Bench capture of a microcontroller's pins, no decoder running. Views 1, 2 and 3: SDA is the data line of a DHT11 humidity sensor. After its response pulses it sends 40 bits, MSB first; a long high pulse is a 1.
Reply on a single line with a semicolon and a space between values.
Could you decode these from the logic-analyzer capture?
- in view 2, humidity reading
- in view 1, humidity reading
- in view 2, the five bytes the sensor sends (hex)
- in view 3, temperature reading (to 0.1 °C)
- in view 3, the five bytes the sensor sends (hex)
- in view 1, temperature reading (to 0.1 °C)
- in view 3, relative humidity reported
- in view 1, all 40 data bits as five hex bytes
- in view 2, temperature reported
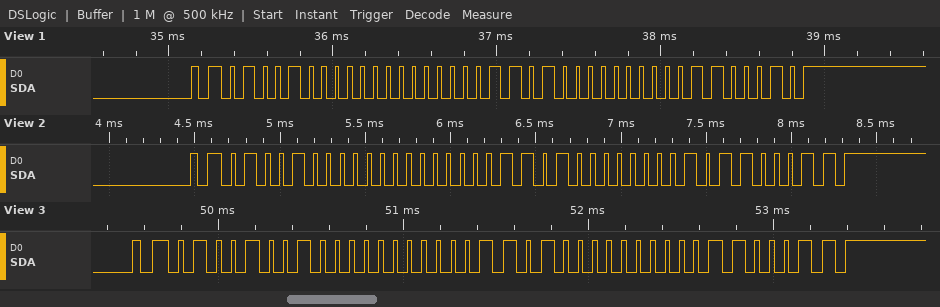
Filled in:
72 %; 72 %; 48 00 1A 01 63; 26.0 °C; 49 00 1A 00 63; 26.0 °C; 73 %; 48 00 1A 00 62; 26.1 °C
